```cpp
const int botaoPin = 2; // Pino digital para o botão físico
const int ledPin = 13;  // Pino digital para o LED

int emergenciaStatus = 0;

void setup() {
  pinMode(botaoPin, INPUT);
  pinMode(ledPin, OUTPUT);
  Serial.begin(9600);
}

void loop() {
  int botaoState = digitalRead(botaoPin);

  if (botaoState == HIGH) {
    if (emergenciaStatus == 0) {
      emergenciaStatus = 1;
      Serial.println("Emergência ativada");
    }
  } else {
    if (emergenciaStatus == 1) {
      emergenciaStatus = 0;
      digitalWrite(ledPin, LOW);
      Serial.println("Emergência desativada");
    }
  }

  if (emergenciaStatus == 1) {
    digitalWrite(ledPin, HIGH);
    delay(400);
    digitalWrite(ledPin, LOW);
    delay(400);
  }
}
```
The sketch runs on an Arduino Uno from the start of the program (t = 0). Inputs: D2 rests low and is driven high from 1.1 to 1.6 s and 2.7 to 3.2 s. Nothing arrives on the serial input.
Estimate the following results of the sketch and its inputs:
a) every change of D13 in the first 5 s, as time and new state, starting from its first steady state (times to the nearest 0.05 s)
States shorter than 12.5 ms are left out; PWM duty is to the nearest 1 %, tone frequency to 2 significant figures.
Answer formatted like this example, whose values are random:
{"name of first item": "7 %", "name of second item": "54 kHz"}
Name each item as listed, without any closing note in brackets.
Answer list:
{"every change of D13 in the first 5 s, as time and new state, starting from its first steady state": "0 s low; 1.1 s high; 1.5 s low; 2.7 s high; 3.1 s low"}
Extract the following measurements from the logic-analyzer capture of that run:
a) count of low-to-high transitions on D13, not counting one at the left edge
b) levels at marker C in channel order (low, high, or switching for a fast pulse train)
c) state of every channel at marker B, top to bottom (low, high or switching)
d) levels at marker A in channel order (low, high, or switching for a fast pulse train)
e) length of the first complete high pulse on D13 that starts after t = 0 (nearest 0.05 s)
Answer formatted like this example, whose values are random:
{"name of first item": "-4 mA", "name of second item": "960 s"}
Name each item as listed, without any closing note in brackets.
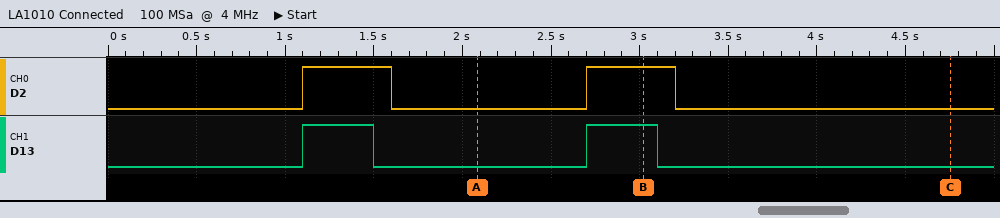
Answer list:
{"count of low-to-high transitions on D13, not counting one at the left edge": "2", "levels at marker C in channel order": "D2 low, D13 low", "state of every channel at marker B, top to bottom": "D2 high, D13 high", "levels at marker A in channel order": "D2 low, D13 low", "length of the first complete high pulse on D13 that starts after t = 0": "0.40 s"}
